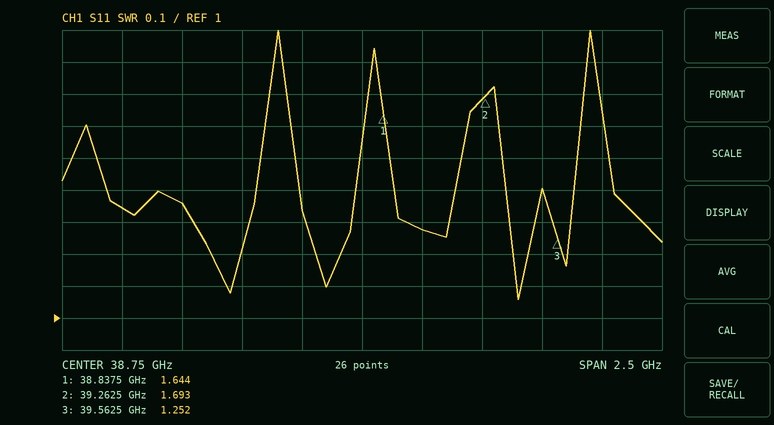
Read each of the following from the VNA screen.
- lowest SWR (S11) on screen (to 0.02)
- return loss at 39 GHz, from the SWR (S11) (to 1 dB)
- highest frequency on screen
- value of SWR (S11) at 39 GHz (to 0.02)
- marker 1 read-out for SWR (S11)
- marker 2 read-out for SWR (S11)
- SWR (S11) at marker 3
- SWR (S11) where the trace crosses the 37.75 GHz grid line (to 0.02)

1.06
18 dB
40 GHz
1.28
1.644
1.693
1.252
1.34
